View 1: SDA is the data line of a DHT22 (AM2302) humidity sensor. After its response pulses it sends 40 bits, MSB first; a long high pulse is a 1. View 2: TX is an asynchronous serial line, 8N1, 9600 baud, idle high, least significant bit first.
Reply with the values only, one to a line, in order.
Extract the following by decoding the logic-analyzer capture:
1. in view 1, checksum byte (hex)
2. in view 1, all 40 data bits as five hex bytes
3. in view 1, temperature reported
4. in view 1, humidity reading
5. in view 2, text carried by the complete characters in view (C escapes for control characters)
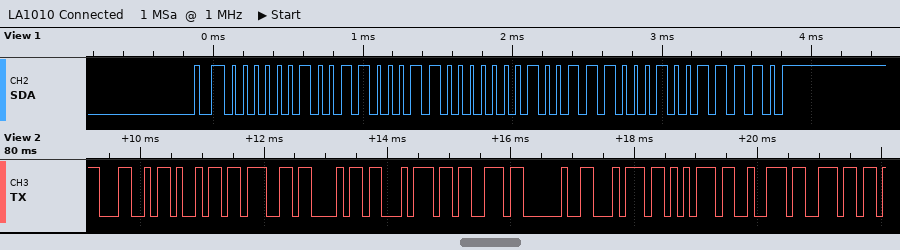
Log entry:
0x9E
02 63 01 38 9E
31.2 °C
61.1 %
"Lights turn"
